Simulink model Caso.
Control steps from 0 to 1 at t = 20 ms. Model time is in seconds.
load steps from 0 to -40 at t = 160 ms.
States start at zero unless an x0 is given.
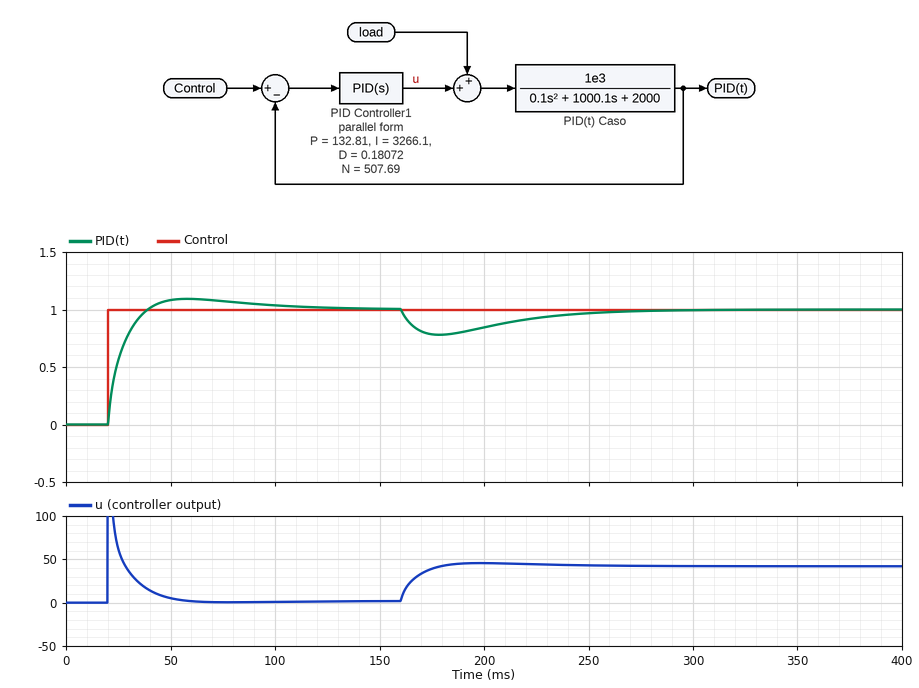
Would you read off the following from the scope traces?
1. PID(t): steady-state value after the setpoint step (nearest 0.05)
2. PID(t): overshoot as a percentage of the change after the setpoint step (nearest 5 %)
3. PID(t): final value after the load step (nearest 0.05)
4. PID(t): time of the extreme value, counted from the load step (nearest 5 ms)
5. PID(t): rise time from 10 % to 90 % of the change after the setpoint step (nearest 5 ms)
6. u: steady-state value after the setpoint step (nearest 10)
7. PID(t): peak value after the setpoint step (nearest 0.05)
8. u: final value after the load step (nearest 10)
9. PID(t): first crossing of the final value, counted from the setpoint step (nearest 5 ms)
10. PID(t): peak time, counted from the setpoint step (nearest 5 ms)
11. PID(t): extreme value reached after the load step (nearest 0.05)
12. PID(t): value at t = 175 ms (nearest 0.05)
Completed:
1.00
10 %
1.00
20 ms
15 ms
0
1.10
40
20 ms
40 ms
0.80
0.80
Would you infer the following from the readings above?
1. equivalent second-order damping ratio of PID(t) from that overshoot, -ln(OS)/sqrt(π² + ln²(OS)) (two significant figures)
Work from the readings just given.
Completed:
0.59
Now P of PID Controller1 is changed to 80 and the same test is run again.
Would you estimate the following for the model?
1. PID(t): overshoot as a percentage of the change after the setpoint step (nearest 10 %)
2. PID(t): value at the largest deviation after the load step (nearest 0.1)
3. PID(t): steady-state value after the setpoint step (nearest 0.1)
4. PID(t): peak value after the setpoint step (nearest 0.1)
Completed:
20 %
0.7
1.0
1.2
